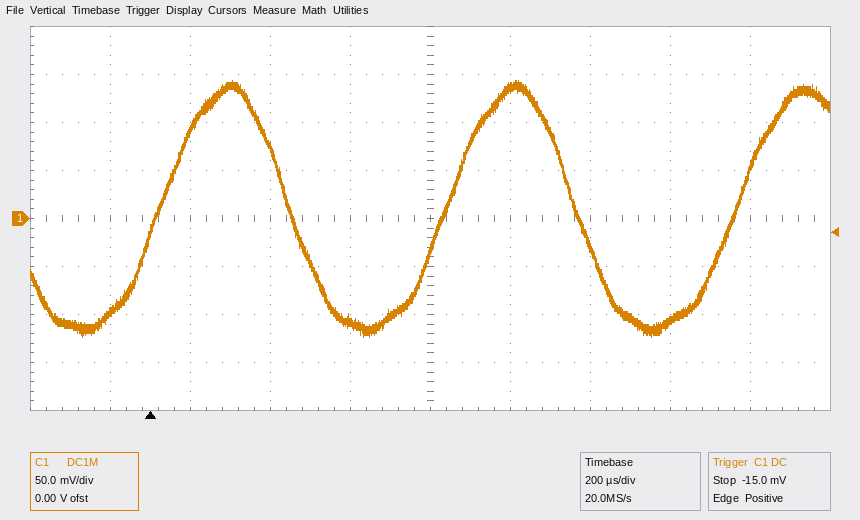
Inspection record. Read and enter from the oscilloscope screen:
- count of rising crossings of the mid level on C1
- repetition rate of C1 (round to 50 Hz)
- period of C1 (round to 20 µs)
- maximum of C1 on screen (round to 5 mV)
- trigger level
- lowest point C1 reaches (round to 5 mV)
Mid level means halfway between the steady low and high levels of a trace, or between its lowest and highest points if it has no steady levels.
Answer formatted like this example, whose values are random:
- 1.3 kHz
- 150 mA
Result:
- 3
- 1.40 kHz
- 720 µs
- 145 mV
- -15.0 mV
- -125 mV
